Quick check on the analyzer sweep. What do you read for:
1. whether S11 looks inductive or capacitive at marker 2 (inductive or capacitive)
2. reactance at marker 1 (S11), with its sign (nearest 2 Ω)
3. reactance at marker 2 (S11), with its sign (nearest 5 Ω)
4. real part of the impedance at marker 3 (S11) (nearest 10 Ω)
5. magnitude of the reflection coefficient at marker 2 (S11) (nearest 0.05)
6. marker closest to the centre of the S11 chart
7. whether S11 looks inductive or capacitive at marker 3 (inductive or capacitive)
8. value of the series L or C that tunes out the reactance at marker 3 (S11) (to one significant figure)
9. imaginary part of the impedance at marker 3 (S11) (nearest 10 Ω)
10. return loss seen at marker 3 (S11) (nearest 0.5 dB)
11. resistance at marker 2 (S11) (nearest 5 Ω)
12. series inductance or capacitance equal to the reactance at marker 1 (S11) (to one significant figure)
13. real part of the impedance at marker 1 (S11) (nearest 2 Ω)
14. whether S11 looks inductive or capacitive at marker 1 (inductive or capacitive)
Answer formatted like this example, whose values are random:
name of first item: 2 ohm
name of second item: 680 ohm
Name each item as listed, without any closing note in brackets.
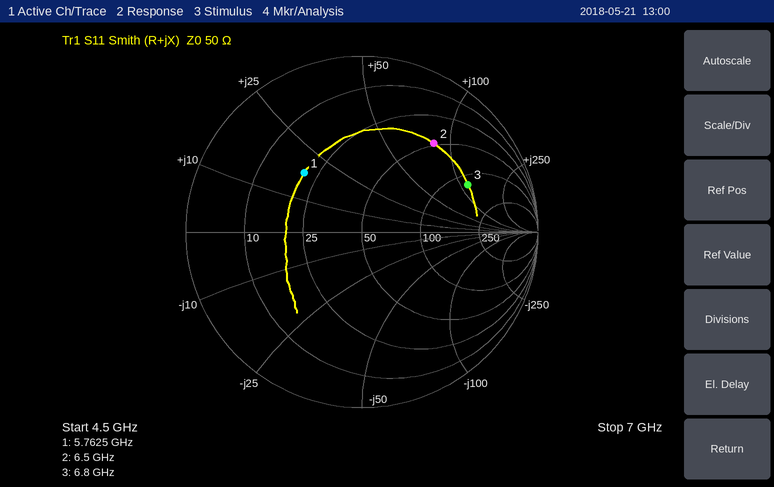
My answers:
whether S11 looks inductive or capacitive at marker 2: inductive
reactance at marker 1 (S11), with its sign: +18 Ω
reactance at marker 2 (S11), with its sign: +85 Ω
real part of the impedance at marker 3 (S11): 120 Ω
magnitude of the reflection coefficient at marker 2 (S11): 0.65
marker closest to the centre of the S11 chart: marker 1
whether S11 looks inductive or capacitive at marker 3: inductive
value of the series L or C that tunes out the reactance at marker 3 (S11): 200 fF
imaginary part of the impedance at marker 3 (S11): +120 Ω
return loss seen at marker 3 (S11): 3.5 dB
resistance at marker 2 (S11): 50 Ω
series inductance or capacitance equal to the reactance at marker 1 (S11): 500 pH
real part of the impedance at marker 1 (S11): 20 Ω
whether S11 looks inductive or capacitive at marker 1: inductive
